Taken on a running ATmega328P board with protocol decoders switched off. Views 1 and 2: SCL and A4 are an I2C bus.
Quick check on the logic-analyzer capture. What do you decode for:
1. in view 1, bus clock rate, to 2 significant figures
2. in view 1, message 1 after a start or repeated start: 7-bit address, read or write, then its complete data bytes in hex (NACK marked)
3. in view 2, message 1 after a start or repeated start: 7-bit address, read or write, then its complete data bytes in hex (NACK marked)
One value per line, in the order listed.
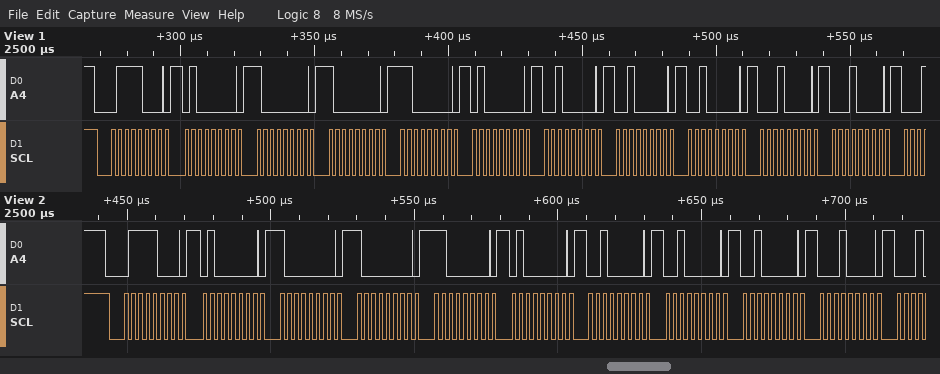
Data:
400 kHz
0x3C write: 40 80 80 C0 40 20 20 20 10 10
0x3C write: 40 80 80 C0 40 20 20 20 10
